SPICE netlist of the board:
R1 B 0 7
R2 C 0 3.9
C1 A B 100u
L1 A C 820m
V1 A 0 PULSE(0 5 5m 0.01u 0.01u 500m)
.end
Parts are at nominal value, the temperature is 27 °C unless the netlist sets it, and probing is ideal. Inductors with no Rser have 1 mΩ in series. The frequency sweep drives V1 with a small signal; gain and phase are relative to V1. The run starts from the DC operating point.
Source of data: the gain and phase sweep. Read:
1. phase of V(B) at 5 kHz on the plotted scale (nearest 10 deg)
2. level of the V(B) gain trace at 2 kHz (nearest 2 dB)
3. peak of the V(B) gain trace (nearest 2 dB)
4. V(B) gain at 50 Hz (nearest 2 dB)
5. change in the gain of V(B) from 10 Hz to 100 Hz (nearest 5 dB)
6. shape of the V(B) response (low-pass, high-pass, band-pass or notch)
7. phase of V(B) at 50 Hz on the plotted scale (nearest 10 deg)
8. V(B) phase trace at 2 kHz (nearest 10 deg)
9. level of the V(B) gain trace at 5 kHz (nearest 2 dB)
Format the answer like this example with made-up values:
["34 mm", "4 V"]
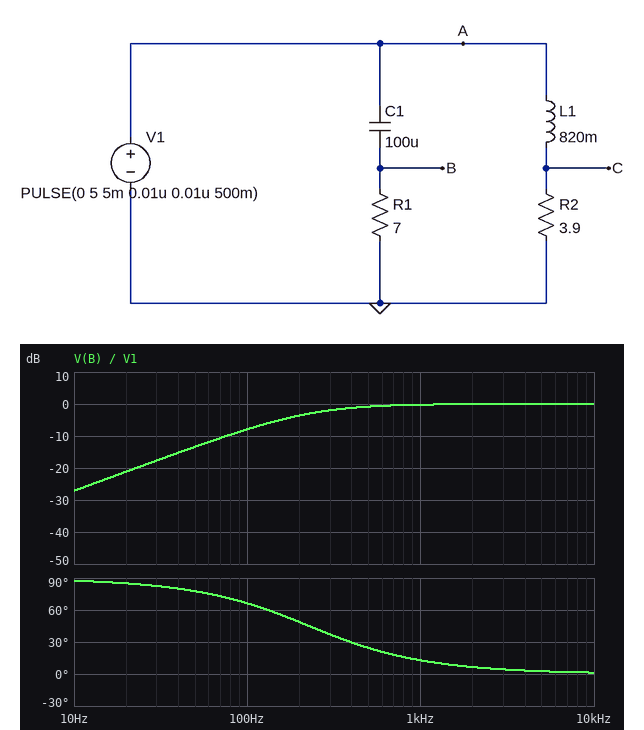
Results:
["0 deg", "0 dB", "0 dB", "-14 dB", "20 dB", "high-pass", "80 deg", "10 deg", "0 dB"]
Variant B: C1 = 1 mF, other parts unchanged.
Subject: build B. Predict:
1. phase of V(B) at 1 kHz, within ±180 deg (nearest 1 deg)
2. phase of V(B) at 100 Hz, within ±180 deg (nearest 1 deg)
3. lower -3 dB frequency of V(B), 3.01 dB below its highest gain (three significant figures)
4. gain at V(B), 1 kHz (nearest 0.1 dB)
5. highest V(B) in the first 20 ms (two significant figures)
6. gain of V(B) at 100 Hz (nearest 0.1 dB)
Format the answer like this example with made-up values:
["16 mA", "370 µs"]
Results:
["1 deg", "13 deg", "22.7 Hz", "0 dB", "5.0 V", "-0.2 dB"]
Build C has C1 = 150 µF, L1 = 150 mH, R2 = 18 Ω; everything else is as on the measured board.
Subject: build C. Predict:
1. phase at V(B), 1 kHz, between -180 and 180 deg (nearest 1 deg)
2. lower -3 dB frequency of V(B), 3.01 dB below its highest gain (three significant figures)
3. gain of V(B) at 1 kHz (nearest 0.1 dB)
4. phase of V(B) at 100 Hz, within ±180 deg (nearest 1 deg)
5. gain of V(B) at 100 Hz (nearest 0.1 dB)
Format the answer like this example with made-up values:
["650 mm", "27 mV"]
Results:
["9 deg", "152 Hz", "-0.1 dB", "57 deg", "-5.2 dB"]
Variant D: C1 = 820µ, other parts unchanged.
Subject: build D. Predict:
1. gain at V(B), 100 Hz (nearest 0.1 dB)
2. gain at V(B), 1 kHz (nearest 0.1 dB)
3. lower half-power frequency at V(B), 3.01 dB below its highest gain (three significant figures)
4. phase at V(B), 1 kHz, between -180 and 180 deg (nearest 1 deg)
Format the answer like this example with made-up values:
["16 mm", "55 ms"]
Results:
["-0.3 dB", "0 dB", "27.7 Hz", "2 deg"]
